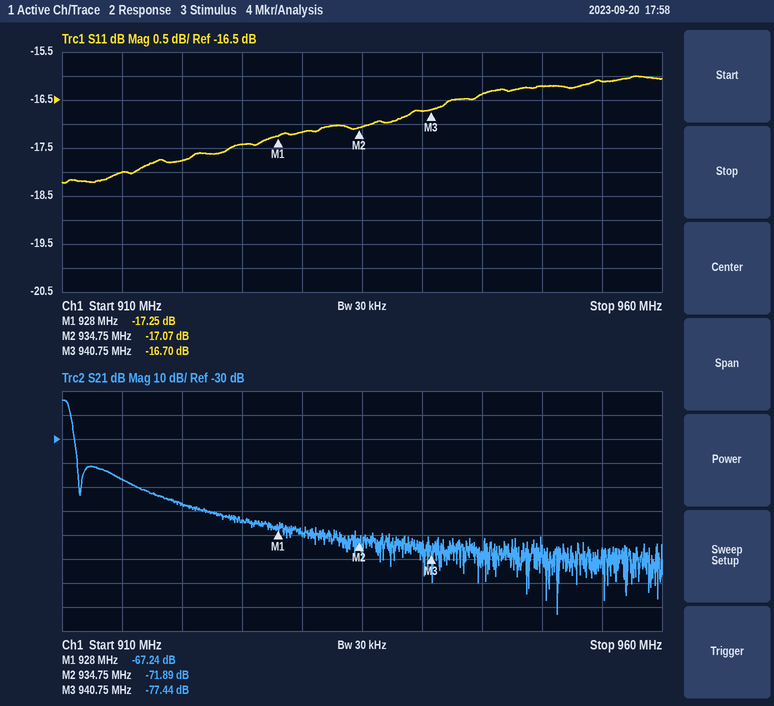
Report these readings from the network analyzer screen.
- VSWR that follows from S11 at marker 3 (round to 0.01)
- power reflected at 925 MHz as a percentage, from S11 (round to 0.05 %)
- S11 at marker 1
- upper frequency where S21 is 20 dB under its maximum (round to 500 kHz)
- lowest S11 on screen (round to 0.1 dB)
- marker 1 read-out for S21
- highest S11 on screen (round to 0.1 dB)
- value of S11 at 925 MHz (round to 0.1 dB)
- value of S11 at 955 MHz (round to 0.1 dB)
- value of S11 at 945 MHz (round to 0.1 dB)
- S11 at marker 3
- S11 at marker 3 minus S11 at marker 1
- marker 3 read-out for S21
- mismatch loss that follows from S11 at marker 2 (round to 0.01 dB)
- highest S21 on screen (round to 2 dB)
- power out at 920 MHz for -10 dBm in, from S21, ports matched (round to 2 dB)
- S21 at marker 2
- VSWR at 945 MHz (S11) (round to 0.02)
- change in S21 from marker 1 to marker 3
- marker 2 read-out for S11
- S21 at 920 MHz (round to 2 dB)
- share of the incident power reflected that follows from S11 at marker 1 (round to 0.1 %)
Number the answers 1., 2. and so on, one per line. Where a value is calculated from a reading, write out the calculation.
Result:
1. (1 + 0.1462)/(1 − 0.1462) ≈ 1.34
2. 10^(-17.4/10) ≈ 1.82 %, so 1.80 % to the nearest 0.05 %
3. -17.25 dB
4. 911.0 MHz
5. -18.2 dB
6. -67.24 dB
7. -16.0 dB
8. -17.4 dB
9. -16.1 dB
10. -16.4 dB
11. -16.70 dB
12. -16.7 − (-17.25) = 0.55 dB
13. -77.44 dB
14. −10 log10(1 − 10^(-17.07/10)) ≈ 0.09 dB
15. -14 dB
16. -10 dBm + (-58 dB) = -68 dBm
17. -71.89 dB
18. |Γ| = 10^(-16.4/20) = 0.1514; VSWR = (1 + 0.1514)/(1 − 0.1514) ≈ 1.36
19. -77.44 − (-67.24) = -10.20 dB
20. -17.07 dB
21. -58 dB
22. 10^(-17.25/10) ≈ 1.9 %
